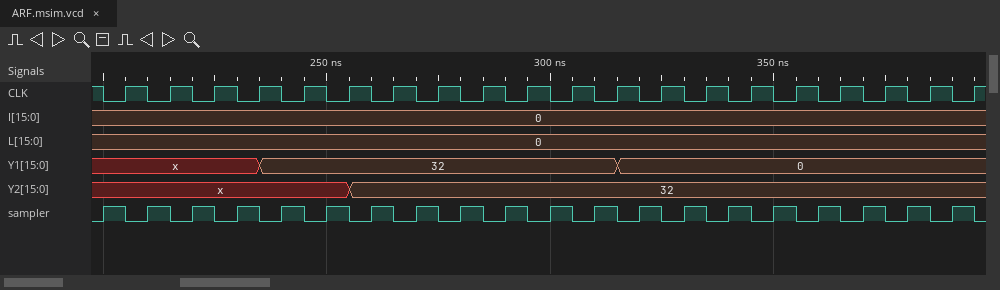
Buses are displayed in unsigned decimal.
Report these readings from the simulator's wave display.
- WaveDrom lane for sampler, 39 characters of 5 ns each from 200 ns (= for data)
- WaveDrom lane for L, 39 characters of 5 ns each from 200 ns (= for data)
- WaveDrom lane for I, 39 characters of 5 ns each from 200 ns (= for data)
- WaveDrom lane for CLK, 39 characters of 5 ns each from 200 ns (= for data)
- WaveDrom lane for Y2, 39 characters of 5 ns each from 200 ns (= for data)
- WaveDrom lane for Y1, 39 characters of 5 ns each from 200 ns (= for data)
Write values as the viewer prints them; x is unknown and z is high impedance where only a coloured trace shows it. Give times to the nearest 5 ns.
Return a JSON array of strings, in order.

["{name: 'sampler', wave: '101010101010101010101010101010101010101'}", "{name: 'L', wave: '=......................................', data: '0'}", "{name: 'I', wave: '=......................................', data: '0'}", "{name: 'CLK', wave: '010101010101010101010101010101010101010'}", "{name: 'Y2', wave: 'x..........=...........................', data: '32'}", "{name: 'Y1', wave: 'x......=...............=...............', data: '32 0'}"]
